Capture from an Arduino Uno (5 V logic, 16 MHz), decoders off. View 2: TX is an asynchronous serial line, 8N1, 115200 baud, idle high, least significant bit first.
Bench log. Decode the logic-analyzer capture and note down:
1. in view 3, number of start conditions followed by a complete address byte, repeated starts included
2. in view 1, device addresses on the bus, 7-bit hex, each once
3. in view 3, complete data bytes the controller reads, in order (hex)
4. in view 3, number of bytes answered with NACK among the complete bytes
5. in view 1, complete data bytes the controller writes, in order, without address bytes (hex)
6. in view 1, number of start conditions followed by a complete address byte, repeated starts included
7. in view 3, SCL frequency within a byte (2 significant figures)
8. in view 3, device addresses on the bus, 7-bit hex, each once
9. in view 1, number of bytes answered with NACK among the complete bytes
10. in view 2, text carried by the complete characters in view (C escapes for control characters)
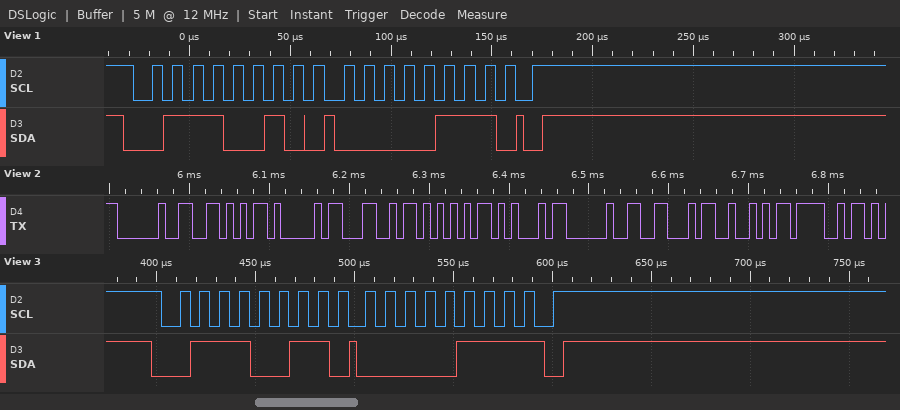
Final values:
1
0x39
07
1
07
1
100 kHz
0x39
0
" VALUE FRO"
